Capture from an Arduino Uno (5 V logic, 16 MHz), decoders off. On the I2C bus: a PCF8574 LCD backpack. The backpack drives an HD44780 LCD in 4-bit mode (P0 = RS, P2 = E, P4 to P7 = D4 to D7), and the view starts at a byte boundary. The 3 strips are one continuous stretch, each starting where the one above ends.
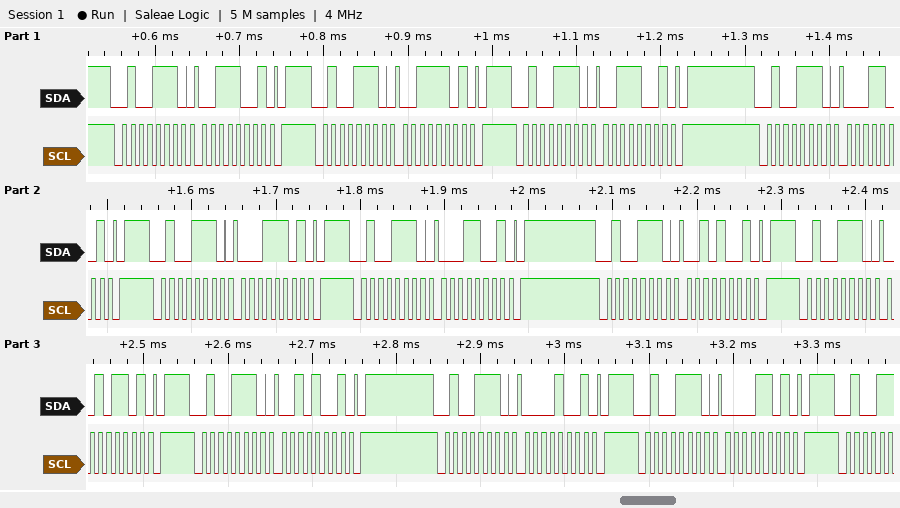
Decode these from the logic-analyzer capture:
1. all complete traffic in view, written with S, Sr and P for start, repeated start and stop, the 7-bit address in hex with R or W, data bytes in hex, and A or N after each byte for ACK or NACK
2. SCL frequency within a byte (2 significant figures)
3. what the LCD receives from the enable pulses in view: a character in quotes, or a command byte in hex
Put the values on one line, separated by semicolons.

S 27W A 39 A P S 27W A 3D A P S 27W A 39 A P S 27W A 19 A P S 27W A 1D A P S 27W A 19 A P S 27W A 29 A P S 27W A 2D A P S 27W A 29 A P S 27W A 09 A P S 27W A 0D A P; 100 kHz; '1'
